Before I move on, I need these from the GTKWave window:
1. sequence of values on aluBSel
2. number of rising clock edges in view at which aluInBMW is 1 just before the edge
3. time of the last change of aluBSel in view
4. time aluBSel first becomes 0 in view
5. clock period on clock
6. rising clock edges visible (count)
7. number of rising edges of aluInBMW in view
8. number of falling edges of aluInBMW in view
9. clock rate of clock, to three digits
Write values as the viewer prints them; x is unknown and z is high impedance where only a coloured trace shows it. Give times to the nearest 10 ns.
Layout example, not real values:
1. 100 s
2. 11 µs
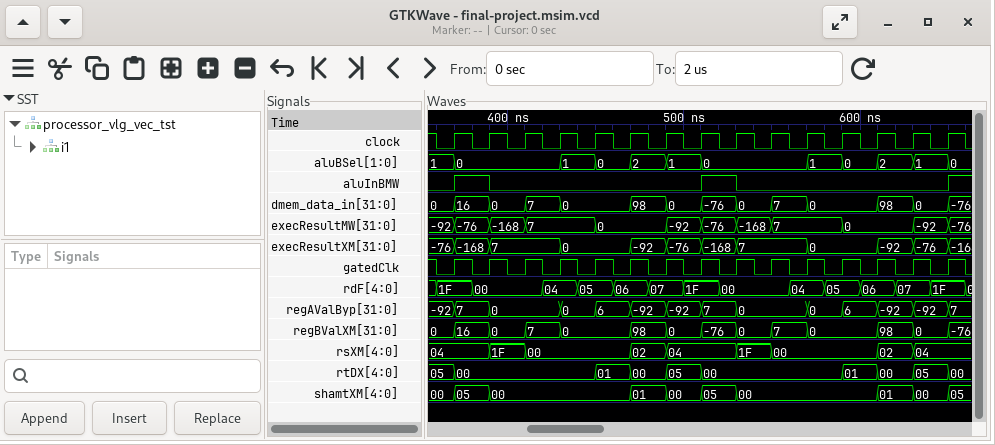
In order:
1. 1, 0, 1, 0, 2, 1, 0, 1, 0, 2, 1, 0
2. 2
3. 650 ns
4. 370 ns
5. 20 ns
6. 15
7. 3
8. 2
9. 50.0 MHz
